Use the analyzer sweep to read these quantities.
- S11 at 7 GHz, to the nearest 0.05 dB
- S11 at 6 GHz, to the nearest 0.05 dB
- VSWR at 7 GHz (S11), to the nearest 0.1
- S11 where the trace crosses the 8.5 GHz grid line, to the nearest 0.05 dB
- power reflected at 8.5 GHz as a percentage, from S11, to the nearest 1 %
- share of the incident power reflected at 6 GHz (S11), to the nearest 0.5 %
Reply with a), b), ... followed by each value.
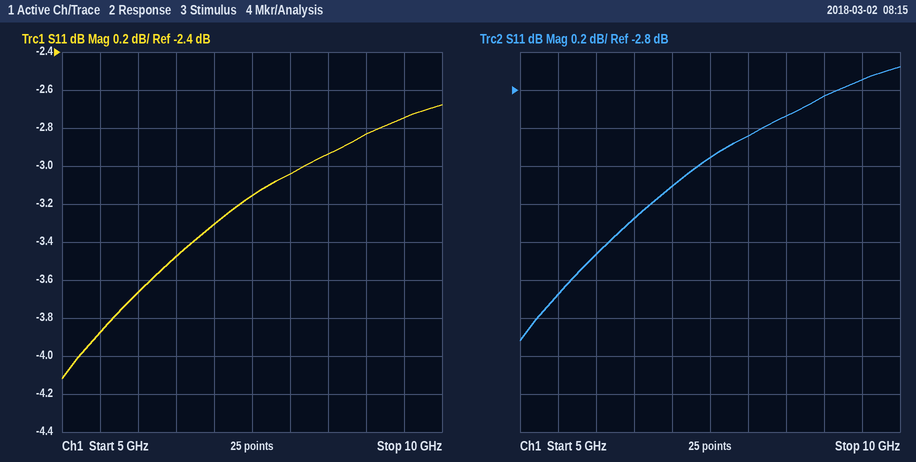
a) -3.30 dB
b) -3.65 dB
c) 5.3
d) -2.95 dB
e) 51 %
f) 43.0 %
